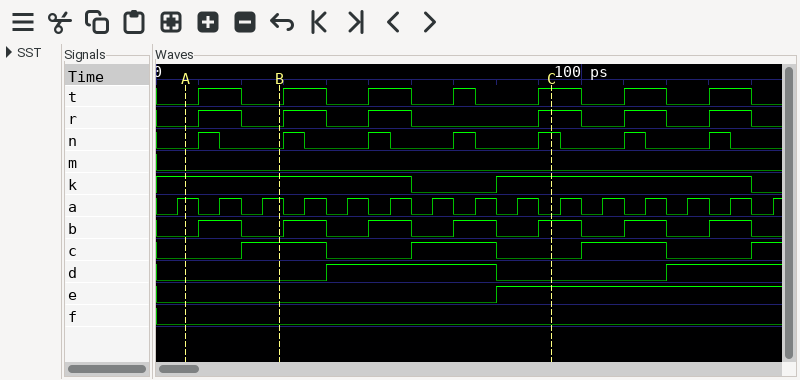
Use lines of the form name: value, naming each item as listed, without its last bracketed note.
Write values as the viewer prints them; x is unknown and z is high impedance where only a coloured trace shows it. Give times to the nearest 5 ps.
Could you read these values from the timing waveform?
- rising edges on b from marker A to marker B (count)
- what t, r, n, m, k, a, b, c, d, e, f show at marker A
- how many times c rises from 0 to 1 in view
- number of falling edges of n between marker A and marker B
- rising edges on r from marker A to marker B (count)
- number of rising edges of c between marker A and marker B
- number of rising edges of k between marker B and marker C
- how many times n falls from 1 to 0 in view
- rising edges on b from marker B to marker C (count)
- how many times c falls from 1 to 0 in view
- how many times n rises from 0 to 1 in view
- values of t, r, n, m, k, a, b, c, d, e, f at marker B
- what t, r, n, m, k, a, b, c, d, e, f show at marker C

rising edges on b from marker A to marker B: 1
what t, r, n, m, k, a, b, c, d, e, f show at marker A: t=0, r=0, n=0, m=0, k=1, a=1, b=0, c=0, d=0, e=0, f=0
how many times c rises from 0 to 1 in view: 4
number of falling edges of n between marker A and marker B: 1
rising edges on r from marker A to marker B: 1
number of rising edges of c between marker A and marker B: 1
number of rising edges of k between marker B and marker C: 1
how many times n falls from 1 to 0 in view: 7
rising edges on b from marker B to marker C: 4
how many times c falls from 1 to 0 in view: 3
how many times n rises from 0 to 1 in view: 7
values of t, r, n, m, k, a, b, c, d, e, f at marker B: t=0, r=0, n=0, m=0, k=1, a=1, b=0, c=1, d=0, e=0, f=0
what t, r, n, m, k, a, b, c, d, e, f show at marker C: t=1, r=1, n=1, m=0, k=1, a=0, b=1, c=0, d=0, e=1, f=0
